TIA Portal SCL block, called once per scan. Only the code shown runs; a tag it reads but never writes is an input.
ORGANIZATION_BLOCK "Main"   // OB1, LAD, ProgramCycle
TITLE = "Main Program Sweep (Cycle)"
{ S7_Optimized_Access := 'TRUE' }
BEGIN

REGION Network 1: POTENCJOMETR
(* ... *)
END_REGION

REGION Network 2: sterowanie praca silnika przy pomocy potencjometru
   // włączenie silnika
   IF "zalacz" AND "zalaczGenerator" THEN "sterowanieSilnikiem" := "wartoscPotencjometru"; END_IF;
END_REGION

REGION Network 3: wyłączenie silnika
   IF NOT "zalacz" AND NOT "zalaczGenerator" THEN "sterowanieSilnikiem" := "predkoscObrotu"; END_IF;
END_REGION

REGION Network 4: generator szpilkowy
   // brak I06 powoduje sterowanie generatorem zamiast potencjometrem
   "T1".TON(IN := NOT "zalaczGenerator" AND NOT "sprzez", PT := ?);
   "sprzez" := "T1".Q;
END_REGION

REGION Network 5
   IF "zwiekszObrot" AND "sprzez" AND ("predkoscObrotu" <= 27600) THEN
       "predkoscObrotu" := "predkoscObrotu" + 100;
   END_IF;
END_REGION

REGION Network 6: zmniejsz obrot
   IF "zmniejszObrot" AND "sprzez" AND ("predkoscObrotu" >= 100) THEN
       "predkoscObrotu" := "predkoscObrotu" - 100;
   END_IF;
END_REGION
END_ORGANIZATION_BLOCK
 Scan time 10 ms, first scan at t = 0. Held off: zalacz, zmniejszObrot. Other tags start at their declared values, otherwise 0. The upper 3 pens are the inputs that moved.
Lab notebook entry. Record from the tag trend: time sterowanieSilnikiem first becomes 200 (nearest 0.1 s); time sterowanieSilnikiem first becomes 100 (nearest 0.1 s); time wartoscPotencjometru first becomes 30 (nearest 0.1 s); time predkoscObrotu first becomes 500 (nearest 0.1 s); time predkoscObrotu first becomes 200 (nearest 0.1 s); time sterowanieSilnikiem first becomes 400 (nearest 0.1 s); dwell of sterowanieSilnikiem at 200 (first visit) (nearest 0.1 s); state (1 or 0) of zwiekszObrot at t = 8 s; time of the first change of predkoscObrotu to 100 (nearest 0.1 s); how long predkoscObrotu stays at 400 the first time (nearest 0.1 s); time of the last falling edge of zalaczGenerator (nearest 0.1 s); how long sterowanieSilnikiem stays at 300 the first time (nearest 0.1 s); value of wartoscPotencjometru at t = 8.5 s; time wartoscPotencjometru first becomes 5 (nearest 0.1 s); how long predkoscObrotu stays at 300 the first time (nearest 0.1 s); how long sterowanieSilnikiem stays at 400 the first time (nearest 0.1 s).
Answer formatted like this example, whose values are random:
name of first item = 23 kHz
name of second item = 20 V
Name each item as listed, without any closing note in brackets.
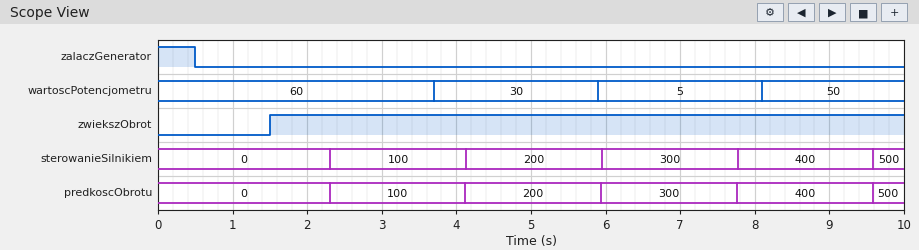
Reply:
time sterowanieSilnikiem first becomes 200 = 4.1 s
time sterowanieSilnikiem first becomes 100 = 2.3 s
time wartoscPotencjometru first becomes 30 = 3.7 s
time predkoscObrotu first becomes 500 = 9.6 s
time predkoscObrotu first becomes 200 = 4.1 s
time sterowanieSilnikiem first becomes 400 = 7.8 s
dwell of sterowanieSilnikiem at 200 (first visit) = 1.8 s
state (1 or 0) of zwiekszObrot at t = 8 s = 1
time of the first change of predkoscObrotu to 100 = 2.3 s
how long predkoscObrotu stays at 400 the first time = 1.8 s
time of the last falling edge of zalaczGenerator = 0.5 s
how long sterowanieSilnikiem stays at 300 the first time = 1.8 s
value of wartoscPotencjometru at t = 8.5 s = 50
time wartoscPotencjometru first becomes 5 = 5.9 s
how long predkoscObrotu stays at 300 the first time = 1.8 s
how long sterowanieSilnikiem stays at 400 the first time = 1.8 s
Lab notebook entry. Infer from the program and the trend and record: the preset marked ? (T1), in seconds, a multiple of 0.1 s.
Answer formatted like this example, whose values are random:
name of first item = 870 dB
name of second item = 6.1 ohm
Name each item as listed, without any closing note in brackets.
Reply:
the preset marked ? (T1), in seconds, a multiple of 0.1 s = 1.8 s
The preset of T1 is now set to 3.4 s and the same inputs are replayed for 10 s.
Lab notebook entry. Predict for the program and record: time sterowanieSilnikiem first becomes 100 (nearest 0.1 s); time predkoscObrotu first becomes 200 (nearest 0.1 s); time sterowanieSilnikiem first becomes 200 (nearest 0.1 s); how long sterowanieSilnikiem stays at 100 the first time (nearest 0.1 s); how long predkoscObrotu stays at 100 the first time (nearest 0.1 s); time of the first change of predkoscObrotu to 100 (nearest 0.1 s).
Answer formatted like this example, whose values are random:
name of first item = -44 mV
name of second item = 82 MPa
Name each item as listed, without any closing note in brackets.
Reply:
time sterowanieSilnikiem first becomes 100 = 3.9 s
time predkoscObrotu first becomes 200 = 7.3 s
time sterowanieSilnikiem first becomes 200 = 7.3 s
how long sterowanieSilnikiem stays at 100 the first time = 3.4 s
how long predkoscObrotu stays at 100 the first time = 3.4 s
time of the first change of predkoscObrotu to 100 = 3.9 s
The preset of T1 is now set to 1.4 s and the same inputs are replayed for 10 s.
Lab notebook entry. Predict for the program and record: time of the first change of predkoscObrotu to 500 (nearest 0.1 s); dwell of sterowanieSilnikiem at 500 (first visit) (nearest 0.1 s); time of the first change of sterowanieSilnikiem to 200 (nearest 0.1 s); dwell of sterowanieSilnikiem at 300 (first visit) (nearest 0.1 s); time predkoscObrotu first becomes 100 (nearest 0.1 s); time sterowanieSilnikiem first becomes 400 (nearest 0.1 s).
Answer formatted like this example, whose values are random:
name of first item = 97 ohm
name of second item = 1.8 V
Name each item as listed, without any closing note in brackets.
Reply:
time of the first change of predkoscObrotu to 500 = 7.6 s
dwell of sterowanieSilnikiem at 500 (first visit) = 1.4 s
time of the first change of sterowanieSilnikiem to 200 = 3.3 s
dwell of sterowanieSilnikiem at 300 (first visit) = 1.4 s
time predkoscObrotu first becomes 100 = 1.9 s
time sterowanieSilnikiem first becomes 400 = 6.2 s
